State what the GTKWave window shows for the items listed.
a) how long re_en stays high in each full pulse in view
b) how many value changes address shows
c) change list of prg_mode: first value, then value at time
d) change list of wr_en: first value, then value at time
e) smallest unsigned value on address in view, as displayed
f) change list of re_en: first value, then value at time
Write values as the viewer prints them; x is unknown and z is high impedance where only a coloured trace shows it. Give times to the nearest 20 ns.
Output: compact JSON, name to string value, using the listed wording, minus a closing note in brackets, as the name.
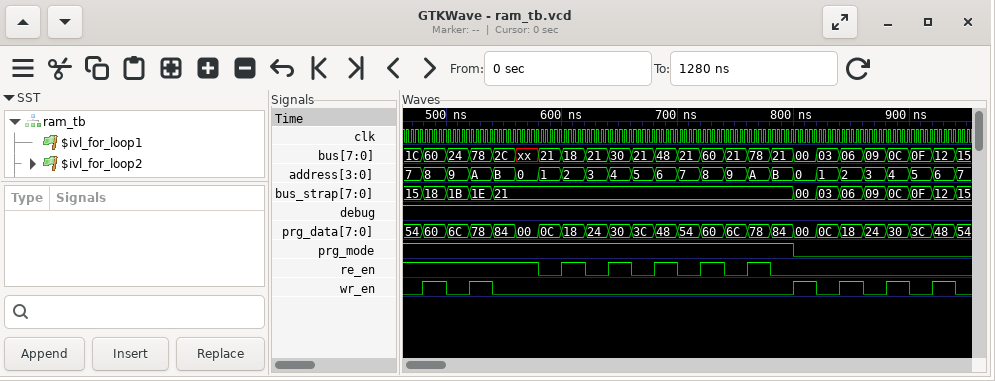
{"how long re_en stays high in each full pulse in view": "20 ns, 20 ns, 20 ns, 20 ns, 20 ns", "how many value changes address shows": "24", "change list of prg_mode: first value, then value at time": "1, 0 at 800 ns", "change list of wr_en: first value, then value at time": "0, 1 at 480 ns, 0 at 500 ns, 1 at 520 ns, 0 at 540 ns, 1 at 800 ns, 0 at 820 ns, 1 at 840 ns, 0 at 860 ns, 1 at 880 ns, 0 at 900 ns, 1 at 920 ns, 0 at 940 ns", "smallest unsigned value on address in view, as displayed": "0", "change list of re_en: first value, then value at time": "1, 0 at 580 ns, 1 at 600 ns, 0 at 620 ns, 1 at 640 ns, 0 at 660 ns, 1 at 680 ns, 0 at 700 ns, 1 at 720 ns, 0 at 740 ns, 1 at 760 ns, 0 at 780 ns"}
